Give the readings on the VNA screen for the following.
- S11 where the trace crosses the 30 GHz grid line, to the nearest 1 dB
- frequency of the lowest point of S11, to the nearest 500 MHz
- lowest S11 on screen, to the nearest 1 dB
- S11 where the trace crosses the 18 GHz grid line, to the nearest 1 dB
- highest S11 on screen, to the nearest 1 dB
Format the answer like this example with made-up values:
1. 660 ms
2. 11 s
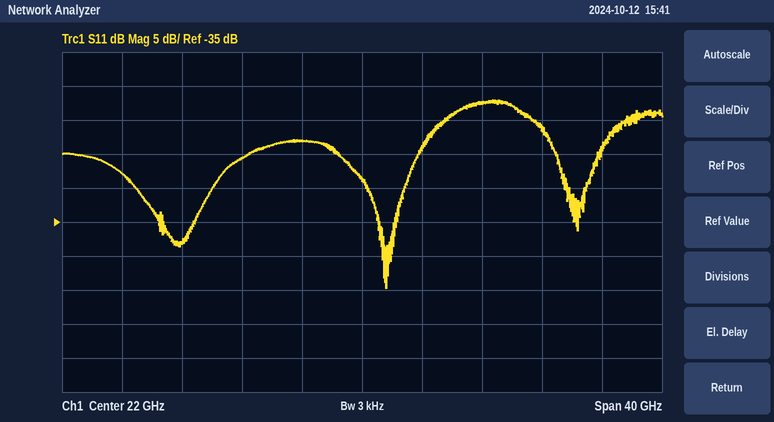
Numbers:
1. -17 dB
2. 23.5 GHz
3. -45 dB
4. -23 dB
5. -17 dB
